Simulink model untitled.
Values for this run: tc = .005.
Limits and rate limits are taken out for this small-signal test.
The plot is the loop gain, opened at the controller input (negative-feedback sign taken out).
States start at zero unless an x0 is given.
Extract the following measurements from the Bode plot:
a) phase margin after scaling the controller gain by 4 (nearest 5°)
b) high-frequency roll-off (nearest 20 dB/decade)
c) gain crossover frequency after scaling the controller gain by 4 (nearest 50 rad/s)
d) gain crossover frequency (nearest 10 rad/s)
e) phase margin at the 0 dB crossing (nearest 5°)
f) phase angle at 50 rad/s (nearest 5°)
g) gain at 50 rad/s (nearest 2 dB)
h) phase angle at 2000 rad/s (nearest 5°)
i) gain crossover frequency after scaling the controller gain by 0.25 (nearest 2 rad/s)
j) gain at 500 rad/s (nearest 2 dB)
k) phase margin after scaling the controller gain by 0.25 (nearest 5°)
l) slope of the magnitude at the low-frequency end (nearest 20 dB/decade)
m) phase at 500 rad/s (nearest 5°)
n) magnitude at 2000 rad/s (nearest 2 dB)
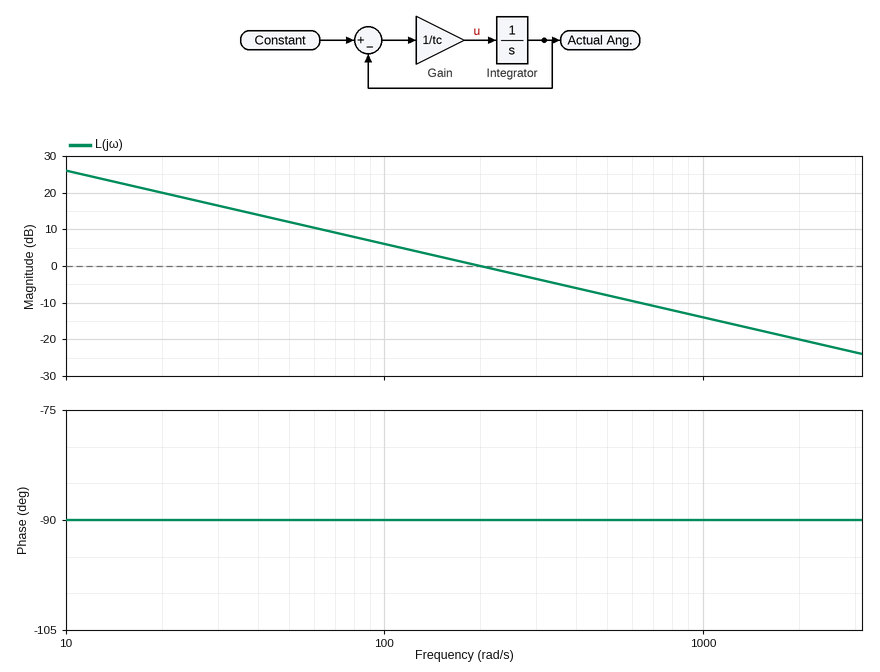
90°
-20 dB/decade
800 rad/s
200 rad/s
90°
-90°
12 dB
-90°
50 rad/s
-8 dB
90°
-20 dB/decade
-90°
-20 dB
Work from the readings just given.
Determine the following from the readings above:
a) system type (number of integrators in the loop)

1
